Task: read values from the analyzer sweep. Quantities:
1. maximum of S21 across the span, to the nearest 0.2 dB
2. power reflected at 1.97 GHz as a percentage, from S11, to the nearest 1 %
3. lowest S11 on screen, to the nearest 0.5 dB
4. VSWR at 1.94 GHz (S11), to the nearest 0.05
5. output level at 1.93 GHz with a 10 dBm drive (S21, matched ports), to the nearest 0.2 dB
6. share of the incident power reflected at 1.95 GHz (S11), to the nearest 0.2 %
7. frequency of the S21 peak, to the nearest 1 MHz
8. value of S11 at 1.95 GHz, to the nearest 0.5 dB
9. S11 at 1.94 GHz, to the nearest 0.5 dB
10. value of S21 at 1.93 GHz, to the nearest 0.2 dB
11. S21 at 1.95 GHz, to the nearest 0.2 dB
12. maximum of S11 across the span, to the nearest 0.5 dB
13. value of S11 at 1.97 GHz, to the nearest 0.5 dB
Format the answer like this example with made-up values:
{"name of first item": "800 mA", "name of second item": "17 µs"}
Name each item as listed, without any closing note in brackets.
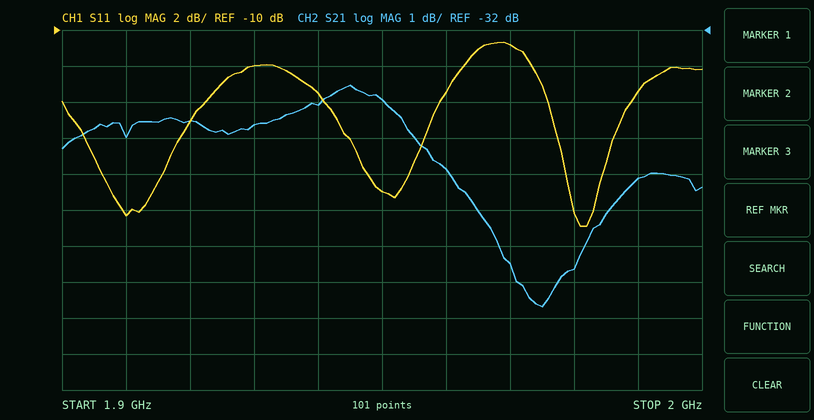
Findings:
{"maximum of S21 across the span, to the nearest 0.2 dB": "-33.6 dB", "power reflected at 1.97 GHz as a percentage, from S11, to the nearest 1 %": "8 %", "lowest S11 on screen, to the nearest 0.5 dB": "-21.0 dB", "VSWR at 1.94 GHz (S11), to the nearest 0.05": "1.55", "output level at 1.93 GHz with a 10 dBm drive (S21, matched ports), to the nearest 0.2 dB": "-24.6 dBm", "share of the incident power reflected at 1.95 GHz (S11), to the nearest 0.2 %": "1.2 %", "frequency of the S21 peak, to the nearest 1 MHz": "1.945 GHz", "value of S11 at 1.95 GHz, to the nearest 0.5 dB": "-19.0 dB", "S11 at 1.94 GHz, to the nearest 0.5 dB": "-13.5 dB", "value of S21 at 1.93 GHz, to the nearest 0.2 dB": "-34.6 dB", "S21 at 1.95 GHz, to the nearest 0.2 dB": "-34.0 dB", "maximum of S11 across the span, to the nearest 0.5 dB": "-10.5 dB", "value of S11 at 1.97 GHz, to the nearest 0.5 dB": "-11.0 dB"}
